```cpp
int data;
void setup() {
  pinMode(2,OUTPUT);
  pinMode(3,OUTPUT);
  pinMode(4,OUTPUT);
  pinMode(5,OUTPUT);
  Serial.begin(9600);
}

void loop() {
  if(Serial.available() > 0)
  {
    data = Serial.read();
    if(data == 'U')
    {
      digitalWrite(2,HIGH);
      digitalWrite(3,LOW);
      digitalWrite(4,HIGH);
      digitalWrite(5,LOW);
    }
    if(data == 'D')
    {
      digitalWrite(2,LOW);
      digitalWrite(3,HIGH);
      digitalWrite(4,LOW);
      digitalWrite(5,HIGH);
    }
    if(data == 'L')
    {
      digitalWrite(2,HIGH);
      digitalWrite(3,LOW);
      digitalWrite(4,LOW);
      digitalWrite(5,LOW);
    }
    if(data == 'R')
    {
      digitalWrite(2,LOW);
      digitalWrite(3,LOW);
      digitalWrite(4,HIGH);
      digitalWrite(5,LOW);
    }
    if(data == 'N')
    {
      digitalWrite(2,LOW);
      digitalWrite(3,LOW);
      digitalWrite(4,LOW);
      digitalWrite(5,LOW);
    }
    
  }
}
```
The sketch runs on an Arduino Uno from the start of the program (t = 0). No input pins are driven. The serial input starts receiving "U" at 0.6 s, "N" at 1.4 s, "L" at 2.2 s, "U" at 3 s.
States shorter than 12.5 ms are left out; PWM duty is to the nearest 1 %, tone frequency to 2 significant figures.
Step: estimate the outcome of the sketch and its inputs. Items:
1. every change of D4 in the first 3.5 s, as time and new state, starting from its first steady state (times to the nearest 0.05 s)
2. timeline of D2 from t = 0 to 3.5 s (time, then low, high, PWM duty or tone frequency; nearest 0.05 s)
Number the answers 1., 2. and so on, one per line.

1. 0 s low; 0.6 s high; 1.4 s low; 3 s high
2. 0 s low; 0.6 s high; 1.4 s low; 2.2 s high
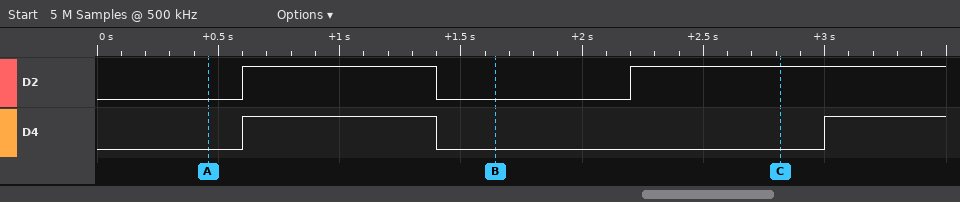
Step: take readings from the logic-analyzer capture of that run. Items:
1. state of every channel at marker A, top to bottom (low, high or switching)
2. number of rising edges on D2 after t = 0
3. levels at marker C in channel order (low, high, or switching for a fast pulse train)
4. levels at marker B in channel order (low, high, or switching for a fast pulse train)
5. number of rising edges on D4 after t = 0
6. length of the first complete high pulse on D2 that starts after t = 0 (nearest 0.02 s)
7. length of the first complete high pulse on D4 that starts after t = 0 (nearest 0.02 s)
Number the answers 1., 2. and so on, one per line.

1. D2 low, D4 low
2. 2
3. D2 high, D4 low
4. D2 low, D4 low
5. 2
6. 0.80 s
7. 0.80 s
